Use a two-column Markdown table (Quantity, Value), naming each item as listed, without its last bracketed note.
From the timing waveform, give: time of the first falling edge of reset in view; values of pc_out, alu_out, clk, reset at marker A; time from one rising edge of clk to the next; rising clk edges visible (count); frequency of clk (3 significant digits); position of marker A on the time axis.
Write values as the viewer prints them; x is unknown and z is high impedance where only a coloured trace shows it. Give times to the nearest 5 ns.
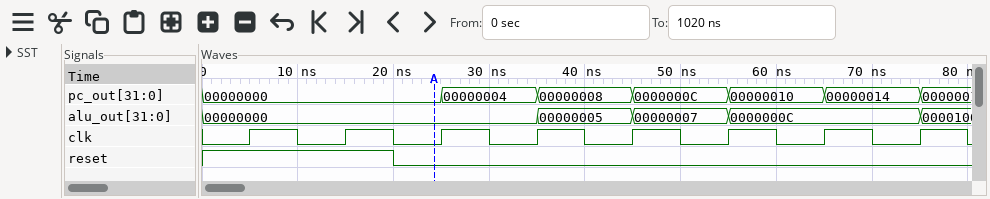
| Quantity | Value |
|---|---|
| time of the first falling edge of reset in view | 20 ns |
| values of pc_out, alu_out, clk, reset at marker A | pc_out=00000000, alu_out=00000000, clk=0, reset=0 |
| time from one rising edge of clk to the next | 10 ns |
| rising clk edges visible | 8 |
| frequency of clk | 100 MHz |
| position of marker A on the time axis | 25 ns |
